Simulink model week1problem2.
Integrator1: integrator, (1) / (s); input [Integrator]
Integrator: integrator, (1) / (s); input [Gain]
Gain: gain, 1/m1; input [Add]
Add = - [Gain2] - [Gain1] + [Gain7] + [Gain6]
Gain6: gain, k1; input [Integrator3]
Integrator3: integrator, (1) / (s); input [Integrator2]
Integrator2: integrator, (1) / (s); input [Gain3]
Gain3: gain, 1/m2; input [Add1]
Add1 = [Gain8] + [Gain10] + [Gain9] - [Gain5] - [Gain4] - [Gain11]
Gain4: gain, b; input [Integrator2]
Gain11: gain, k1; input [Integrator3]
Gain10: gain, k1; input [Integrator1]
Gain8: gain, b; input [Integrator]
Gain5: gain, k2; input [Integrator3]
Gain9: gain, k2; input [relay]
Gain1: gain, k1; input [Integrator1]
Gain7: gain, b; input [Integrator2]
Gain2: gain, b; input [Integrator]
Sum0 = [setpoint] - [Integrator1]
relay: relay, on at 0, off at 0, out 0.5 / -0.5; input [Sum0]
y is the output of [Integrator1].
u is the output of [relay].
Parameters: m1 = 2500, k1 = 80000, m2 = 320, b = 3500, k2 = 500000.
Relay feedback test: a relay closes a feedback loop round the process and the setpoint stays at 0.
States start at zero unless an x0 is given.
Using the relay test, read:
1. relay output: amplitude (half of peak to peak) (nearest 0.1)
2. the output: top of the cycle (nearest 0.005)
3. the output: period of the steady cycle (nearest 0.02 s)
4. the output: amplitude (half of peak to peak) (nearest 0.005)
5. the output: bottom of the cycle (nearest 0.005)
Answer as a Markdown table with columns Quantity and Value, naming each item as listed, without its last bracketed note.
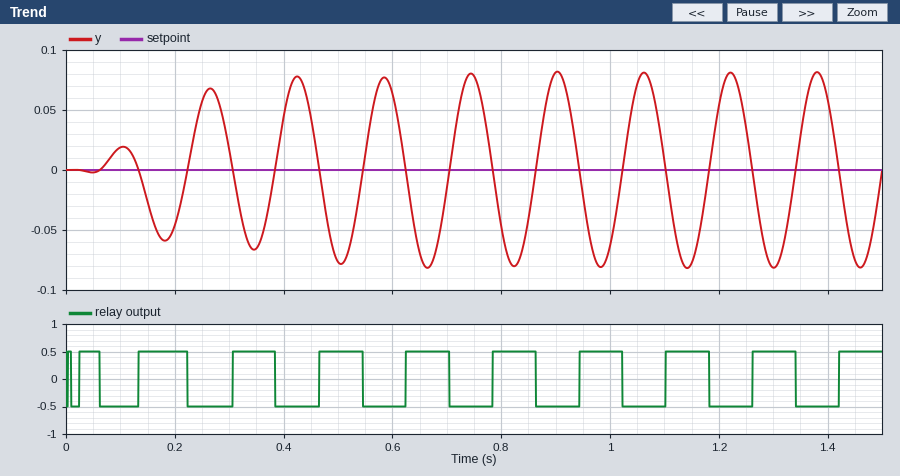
| Quantity | Value |
|---|---|
| relay output: amplitude (half of peak to peak) | 0.5 |
| the output: top of the cycle | 0.080 |
| the output: period of the steady cycle | 0.16 s |
| the output: amplitude (half of peak to peak) | 0.080 |
| the output: bottom of the cycle | -0.080 |
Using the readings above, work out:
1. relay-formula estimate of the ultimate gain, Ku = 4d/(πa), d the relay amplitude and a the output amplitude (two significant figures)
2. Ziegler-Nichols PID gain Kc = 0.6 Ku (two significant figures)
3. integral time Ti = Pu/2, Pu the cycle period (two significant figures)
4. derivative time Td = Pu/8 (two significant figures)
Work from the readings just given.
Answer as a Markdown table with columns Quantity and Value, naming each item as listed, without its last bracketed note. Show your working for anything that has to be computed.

| Quantity | Value |
|---|---|
| relay-formula estimate of the ultimate gain, Ku = 4d/(πa), d the relay amplitude and a the output amplitude | 4 × 0.5 / (π × 0.08) = 8.0 |
| Ziegler-Nichols PID gain Kc = 0.6 Ku | 0.6 × 8 = 4.8 |
| integral time Ti = Pu/2, Pu the cycle period | 0.16 / 2 = 0.080 s |
| derivative time Td = Pu/8 | 0.16 / 8 = 0.020 s |
